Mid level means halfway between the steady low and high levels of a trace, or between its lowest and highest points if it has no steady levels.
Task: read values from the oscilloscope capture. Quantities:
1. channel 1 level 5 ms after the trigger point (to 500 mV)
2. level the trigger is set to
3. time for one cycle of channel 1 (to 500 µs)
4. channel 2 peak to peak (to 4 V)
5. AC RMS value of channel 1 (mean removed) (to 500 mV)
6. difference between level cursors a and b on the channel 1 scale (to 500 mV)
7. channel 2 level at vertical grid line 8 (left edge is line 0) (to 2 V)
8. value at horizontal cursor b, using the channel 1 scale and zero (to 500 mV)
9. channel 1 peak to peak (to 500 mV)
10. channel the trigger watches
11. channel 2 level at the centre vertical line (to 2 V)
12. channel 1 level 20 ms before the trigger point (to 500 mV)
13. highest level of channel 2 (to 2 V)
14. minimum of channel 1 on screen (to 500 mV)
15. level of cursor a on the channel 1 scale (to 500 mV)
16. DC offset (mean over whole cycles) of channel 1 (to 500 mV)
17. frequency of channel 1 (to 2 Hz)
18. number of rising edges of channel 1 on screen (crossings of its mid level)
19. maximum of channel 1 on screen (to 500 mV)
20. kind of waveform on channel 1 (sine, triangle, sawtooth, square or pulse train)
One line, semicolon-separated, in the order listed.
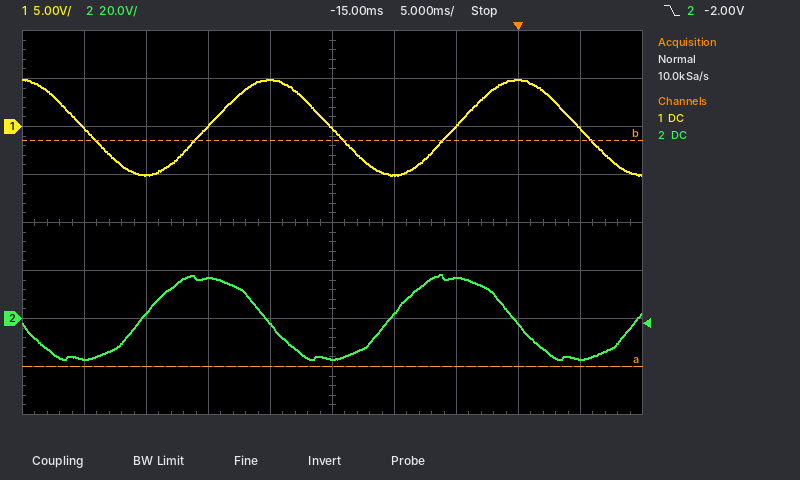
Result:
0.0 V; -2.00 V; 20.0 ms; 36 V; 3.5 V; 23.5 V; -2 V; -1.5 V; 10.0 V; channel 2; -16 V; 5.0 V; 18 V; -5.0 V; -25.0 V; 0.0 V; 50 Hz; 2; 5.0 V; sine
